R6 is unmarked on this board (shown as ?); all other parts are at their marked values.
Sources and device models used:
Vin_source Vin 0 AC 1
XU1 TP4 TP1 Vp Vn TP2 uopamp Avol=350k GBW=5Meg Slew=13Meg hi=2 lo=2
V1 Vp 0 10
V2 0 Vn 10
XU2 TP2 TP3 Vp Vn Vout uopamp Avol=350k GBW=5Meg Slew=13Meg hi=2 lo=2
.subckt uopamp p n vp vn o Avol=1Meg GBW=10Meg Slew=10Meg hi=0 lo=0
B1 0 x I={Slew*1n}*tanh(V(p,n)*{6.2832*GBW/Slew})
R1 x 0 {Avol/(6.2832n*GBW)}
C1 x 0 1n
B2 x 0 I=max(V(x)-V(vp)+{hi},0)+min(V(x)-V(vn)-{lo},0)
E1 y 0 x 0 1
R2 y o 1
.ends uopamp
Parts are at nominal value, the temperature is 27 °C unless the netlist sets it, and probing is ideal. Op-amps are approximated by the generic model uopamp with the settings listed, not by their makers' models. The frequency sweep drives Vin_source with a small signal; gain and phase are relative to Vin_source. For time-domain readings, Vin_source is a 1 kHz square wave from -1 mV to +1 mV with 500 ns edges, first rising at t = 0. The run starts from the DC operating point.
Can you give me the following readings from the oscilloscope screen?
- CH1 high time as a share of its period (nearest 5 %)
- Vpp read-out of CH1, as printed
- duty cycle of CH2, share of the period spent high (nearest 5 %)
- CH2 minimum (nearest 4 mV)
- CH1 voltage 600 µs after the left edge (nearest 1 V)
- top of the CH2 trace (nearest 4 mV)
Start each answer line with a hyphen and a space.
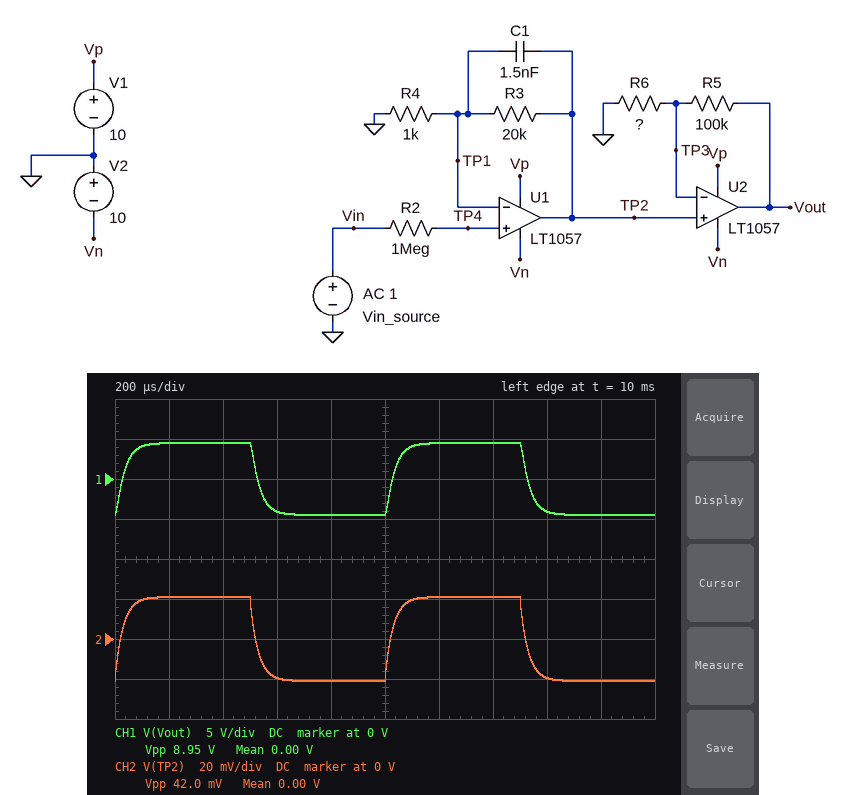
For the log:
- 50 %
- 8.95 V
- 50 %
- -20 mV
- -4 V
- 20 mV
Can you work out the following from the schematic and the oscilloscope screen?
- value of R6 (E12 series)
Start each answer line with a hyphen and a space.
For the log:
- 470 Ω
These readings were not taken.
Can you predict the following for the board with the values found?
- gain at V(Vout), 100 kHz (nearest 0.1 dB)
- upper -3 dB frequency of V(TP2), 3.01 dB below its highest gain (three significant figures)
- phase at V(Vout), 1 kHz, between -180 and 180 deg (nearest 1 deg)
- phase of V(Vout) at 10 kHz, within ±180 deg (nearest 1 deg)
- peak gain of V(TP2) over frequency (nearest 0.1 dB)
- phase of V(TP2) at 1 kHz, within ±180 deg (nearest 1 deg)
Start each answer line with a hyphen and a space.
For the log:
- 37.1 dB
- 5.21 kHz
- -13 deg
- -81 deg
- 26.4 dB
- -10 deg
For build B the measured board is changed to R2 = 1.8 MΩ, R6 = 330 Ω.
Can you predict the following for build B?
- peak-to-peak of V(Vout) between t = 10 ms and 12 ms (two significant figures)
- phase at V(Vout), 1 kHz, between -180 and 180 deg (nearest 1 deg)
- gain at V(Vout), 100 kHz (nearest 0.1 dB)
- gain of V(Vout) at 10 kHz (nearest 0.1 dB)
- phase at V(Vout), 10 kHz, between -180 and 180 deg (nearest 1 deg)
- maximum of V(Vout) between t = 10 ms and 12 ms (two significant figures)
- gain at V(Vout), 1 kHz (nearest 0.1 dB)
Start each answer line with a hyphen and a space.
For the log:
- 13 V
- -14 deg
- 37.2 dB
- 68.0 dB
- -89 deg
- 6.4 V
- 75.9 dB
